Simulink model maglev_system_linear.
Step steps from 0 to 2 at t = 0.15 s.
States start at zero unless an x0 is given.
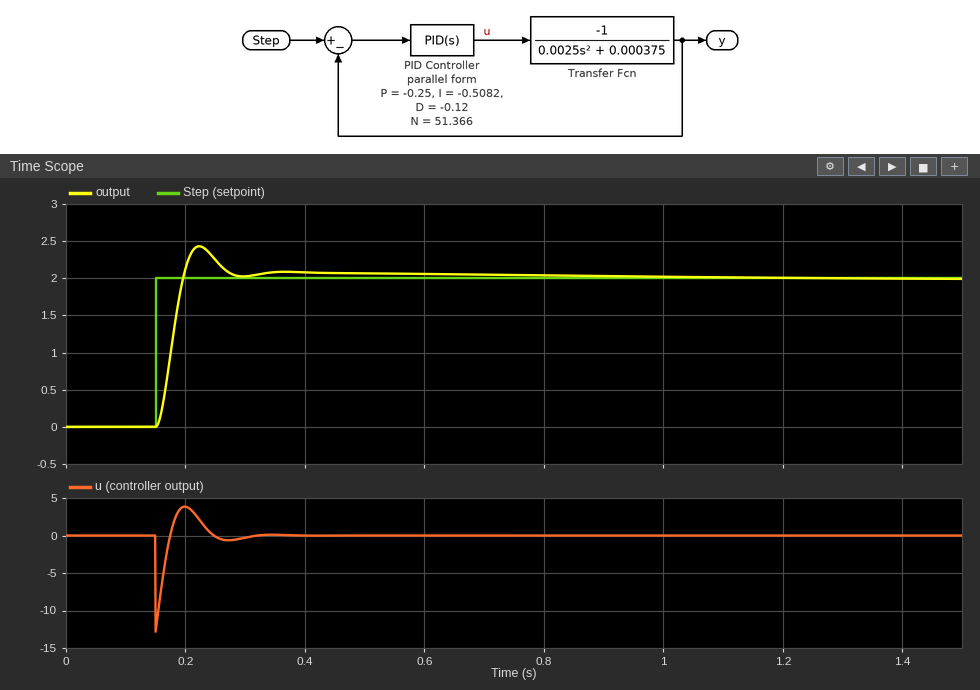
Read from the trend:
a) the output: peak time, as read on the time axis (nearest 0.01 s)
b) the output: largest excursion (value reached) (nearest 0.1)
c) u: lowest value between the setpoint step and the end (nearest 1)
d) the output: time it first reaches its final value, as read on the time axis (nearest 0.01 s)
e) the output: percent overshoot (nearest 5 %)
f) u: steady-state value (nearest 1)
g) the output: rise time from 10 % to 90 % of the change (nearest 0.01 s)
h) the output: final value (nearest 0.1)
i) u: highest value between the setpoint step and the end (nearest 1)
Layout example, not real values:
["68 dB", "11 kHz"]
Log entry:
["0.22 s", "2.4", "-13", "0.20 s", "20 %", "0", "0.03 s", "2.0", "4"]
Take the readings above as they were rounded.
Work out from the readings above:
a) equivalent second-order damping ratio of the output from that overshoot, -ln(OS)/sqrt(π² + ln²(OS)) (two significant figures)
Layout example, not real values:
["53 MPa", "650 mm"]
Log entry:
["0.46"]
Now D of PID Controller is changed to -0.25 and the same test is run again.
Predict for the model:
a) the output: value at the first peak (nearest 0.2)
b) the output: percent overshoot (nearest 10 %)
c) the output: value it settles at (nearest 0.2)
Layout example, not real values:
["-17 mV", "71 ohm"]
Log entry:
["2.6", "30 %", "2.0"]
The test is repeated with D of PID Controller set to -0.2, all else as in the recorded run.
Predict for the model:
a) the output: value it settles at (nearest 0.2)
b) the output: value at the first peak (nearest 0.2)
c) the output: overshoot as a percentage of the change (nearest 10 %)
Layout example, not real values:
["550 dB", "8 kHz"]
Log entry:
["2.0", "2.6", "30 %"]
